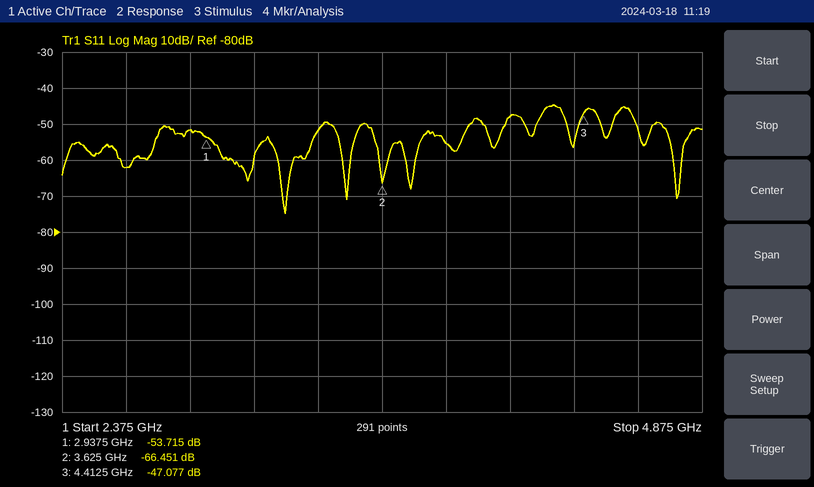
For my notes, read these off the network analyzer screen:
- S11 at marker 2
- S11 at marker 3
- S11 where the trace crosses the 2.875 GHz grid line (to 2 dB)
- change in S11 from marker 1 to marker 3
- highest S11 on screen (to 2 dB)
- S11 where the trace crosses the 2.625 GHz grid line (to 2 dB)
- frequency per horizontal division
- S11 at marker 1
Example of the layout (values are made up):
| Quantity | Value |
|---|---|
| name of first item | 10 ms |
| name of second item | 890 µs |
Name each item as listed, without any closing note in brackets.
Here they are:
| Quantity | Value |
|---|---|
| S11 at marker 2 | -66.451 dB |
| S11 at marker 3 | -47.077 dB |
| S11 where the trace crosses the 2.875 GHz grid line | -52 dB |
| change in S11 from marker 1 to marker 3 | 6.638 dB |
| highest S11 on screen | -44 dB |
| S11 where the trace crosses the 2.625 GHz grid line | -62 dB |
| frequency per horizontal division | 250 MHz |
| S11 at marker 1 | -53.715 dB |
